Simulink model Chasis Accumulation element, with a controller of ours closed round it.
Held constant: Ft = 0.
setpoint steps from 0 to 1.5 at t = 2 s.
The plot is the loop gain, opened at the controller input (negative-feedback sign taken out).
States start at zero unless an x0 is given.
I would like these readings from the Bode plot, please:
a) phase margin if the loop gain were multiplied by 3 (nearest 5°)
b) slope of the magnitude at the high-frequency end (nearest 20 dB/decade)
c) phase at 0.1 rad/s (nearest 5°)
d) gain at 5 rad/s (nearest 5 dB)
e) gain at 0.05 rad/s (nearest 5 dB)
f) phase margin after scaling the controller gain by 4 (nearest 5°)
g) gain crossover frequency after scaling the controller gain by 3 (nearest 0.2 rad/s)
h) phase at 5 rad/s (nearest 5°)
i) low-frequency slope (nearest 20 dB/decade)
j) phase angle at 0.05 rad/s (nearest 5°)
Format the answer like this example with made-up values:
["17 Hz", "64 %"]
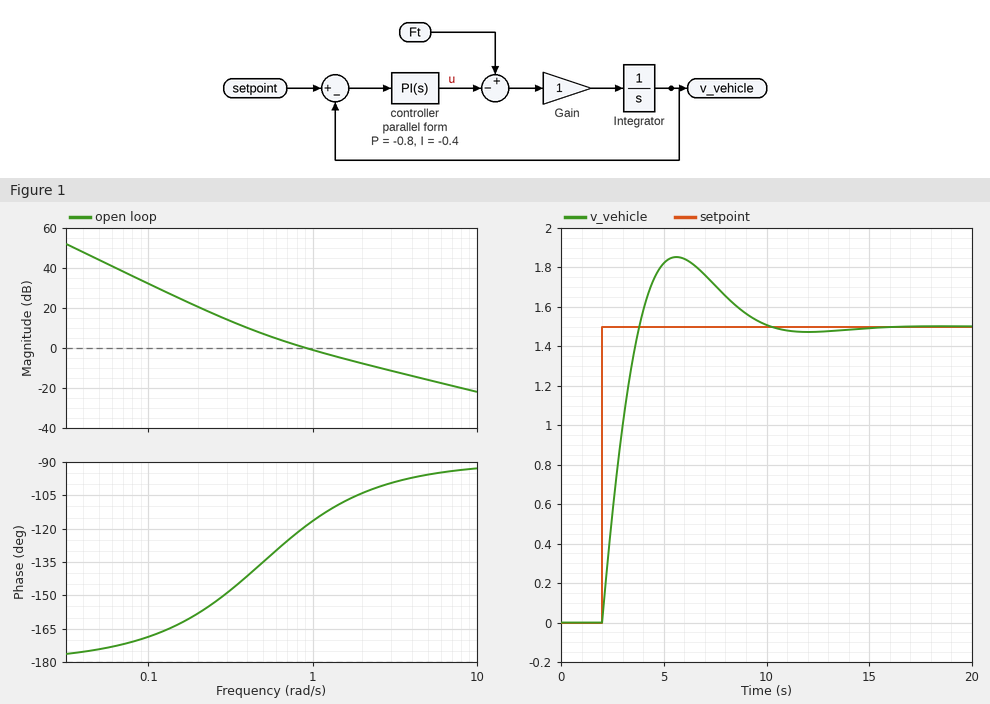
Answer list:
["80°", "-20 dB/decade", "-170°", "-15 dB", "45 dB", "80°", "2.4 rad/s", "-95°", "-40 dB/decade", "-175°"]
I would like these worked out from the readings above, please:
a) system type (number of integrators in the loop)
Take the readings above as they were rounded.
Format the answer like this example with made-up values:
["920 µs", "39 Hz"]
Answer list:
["2"]
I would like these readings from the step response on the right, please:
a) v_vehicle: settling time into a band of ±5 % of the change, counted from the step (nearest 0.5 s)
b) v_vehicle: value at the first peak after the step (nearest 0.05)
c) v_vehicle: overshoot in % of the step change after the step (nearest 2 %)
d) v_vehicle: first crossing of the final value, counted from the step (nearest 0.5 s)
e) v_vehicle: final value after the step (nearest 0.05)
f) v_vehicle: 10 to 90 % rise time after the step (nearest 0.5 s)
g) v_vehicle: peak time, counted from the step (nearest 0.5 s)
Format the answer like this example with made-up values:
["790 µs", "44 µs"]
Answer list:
["7.0 s", "1.85", "24 %", "2.0 s", "1.50", "1.5 s", "3.5 s"]
